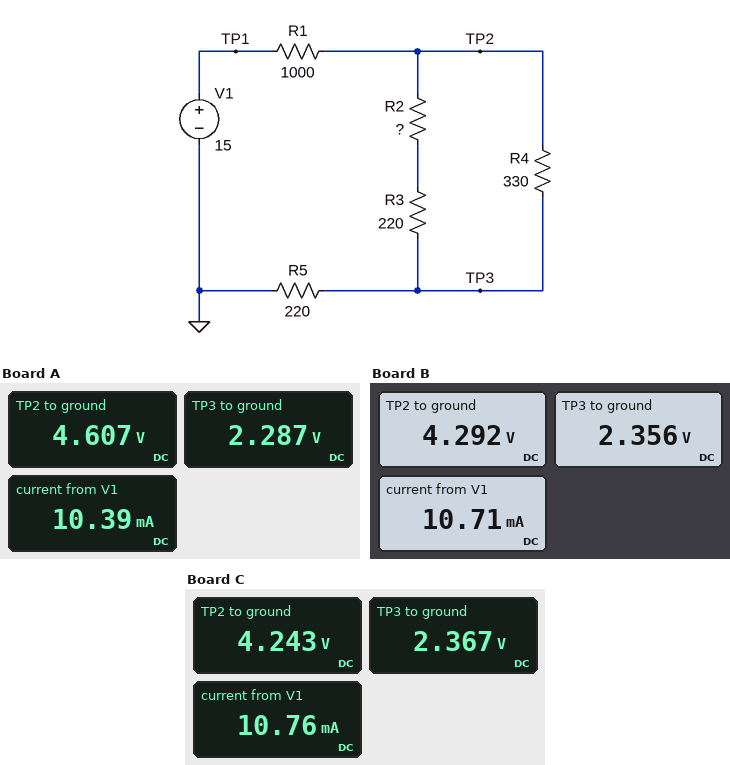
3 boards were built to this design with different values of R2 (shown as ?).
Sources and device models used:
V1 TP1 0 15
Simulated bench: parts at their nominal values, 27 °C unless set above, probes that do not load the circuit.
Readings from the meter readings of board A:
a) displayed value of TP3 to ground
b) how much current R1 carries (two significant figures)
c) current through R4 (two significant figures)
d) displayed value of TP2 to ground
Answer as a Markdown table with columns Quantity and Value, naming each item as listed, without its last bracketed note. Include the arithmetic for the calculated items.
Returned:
| Quantity | Value |
|---|---|
| displayed value of TP3 to ground | 2.287 V |
| how much current R1 carries | (15 V - 4.607 V) / 1 kΩ = 10 mA |
| current through R4 | (4.607 V - 2.287 V) / 330 Ω = 7.0 mA |
| displayed value of TP2 to ground | 4.607 V |
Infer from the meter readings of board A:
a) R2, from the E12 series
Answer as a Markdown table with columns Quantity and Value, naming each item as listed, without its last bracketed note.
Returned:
| Quantity | Value |
|---|---|
| R2, from the E12 series | 470 Ω |
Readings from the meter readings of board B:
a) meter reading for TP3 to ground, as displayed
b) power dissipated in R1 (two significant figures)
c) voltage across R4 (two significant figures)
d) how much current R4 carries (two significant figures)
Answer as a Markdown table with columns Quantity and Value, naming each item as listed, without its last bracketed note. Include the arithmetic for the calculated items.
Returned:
| Quantity | Value |
|---|---|
| meter reading for TP3 to ground, as displayed | 2.356 V |
| power dissipated in R1 | (15 V - 4.292 V)^2 / 1 kΩ = 110 mW |
| voltage across R4 | 4.292 V - 2.356 V = 1.9 V |
| how much current R4 carries | (4.292 V - 2.356 V) / 330 Ω = 5.9 mA |
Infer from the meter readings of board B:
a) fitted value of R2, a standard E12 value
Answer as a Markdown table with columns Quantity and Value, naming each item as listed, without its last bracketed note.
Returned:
| Quantity | Value |
|---|---|
| fitted value of R2, a standard E12 value | 180 Ω |
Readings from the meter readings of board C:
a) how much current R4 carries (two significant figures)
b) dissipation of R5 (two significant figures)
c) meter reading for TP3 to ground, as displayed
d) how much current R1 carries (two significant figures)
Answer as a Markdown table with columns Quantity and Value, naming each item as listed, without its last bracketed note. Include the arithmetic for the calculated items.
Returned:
| Quantity | Value |
|---|---|
| how much current R4 carries | (4.243 V - 2.367 V) / 330 Ω = 5.7 mA |
| dissipation of R5 | (2.367 V)^2 / 220 Ω = 25 mW |
| meter reading for TP3 to ground, as displayed | 2.367 V |
| how much current R1 carries | (15 V - 4.243 V) / 1 kΩ = 11 mA |
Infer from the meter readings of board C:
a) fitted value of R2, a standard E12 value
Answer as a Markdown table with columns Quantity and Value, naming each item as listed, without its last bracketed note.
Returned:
| Quantity | Value |
|---|---|
| fitted value of R2, a standard E12 value | 150 Ω |
